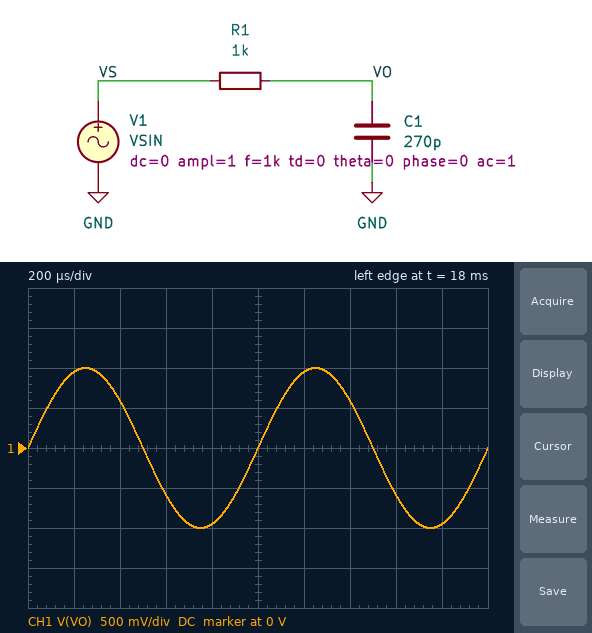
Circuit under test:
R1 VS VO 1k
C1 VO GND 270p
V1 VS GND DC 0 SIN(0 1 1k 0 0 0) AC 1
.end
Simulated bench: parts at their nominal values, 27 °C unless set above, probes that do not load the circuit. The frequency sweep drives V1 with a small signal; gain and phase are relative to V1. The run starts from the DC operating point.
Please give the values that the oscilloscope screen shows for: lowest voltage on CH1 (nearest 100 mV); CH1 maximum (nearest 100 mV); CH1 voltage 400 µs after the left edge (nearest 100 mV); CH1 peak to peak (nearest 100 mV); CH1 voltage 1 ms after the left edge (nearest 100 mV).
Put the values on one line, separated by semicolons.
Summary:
-1.0 V; 1.0 V; 600 mV; 2.0 V; 0 V
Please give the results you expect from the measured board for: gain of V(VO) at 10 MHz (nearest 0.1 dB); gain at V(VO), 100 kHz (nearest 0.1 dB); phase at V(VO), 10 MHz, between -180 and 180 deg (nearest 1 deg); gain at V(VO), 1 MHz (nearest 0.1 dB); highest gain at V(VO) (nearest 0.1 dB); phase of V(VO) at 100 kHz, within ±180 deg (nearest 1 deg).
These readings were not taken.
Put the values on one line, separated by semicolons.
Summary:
-24.6 dB; -0.1 dB; -87 deg; -5.9 dB; 0 dB; -10 deg
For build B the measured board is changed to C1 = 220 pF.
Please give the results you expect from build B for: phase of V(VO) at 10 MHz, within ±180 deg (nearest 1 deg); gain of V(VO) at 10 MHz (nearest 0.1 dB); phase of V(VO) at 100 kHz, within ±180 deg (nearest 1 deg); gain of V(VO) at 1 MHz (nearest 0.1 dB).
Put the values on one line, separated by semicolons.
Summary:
-86 deg; -22.8 dB; -8 deg; -4.6 dB
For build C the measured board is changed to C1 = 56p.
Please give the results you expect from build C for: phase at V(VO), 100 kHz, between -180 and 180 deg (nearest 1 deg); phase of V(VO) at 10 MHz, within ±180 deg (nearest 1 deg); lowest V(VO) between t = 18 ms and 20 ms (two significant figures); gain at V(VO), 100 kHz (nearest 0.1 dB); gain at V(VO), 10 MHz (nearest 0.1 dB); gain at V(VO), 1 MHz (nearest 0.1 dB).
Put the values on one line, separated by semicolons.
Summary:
-2 deg; -74 deg; -1.0 V; 0 dB; -11.3 dB; -0.5 dB
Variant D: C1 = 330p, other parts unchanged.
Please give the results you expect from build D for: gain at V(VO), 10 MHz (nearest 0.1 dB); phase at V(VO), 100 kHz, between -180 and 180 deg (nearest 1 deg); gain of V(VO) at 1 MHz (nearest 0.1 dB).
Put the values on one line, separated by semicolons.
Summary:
-26.3 dB; -12 deg; -7.2 dB
